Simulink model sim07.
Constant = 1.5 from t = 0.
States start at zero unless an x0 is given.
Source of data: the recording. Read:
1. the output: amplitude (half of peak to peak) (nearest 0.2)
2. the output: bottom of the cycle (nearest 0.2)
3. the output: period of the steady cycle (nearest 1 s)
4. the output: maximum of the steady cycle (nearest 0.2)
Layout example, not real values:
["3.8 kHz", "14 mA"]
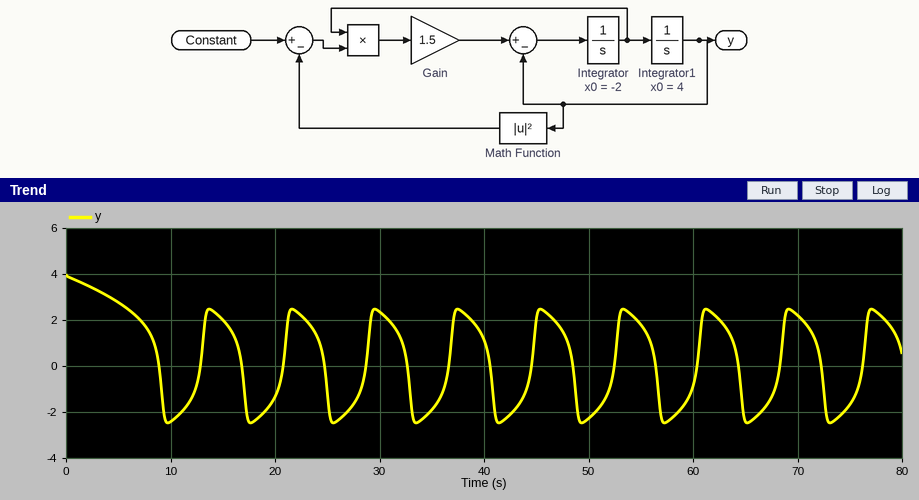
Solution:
["2.4", "-2.4", "8 s", "2.4"]
